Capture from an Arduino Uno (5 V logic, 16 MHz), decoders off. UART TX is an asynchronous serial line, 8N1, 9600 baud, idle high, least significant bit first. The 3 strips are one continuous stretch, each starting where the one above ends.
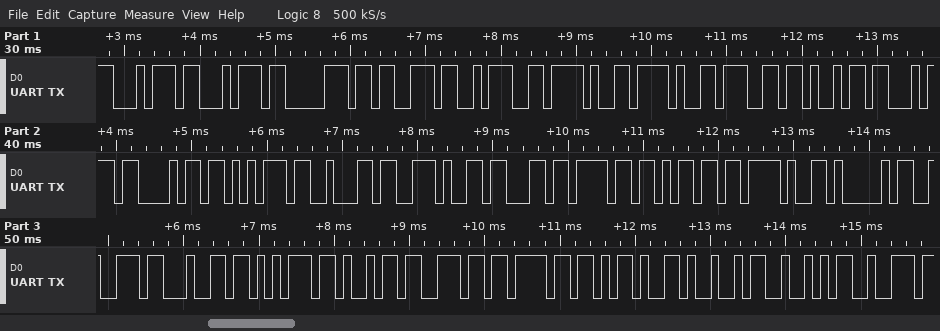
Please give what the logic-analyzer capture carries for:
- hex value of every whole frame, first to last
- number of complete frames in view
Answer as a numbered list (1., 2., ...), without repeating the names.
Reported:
1. 74 74 70 73 3A 2F 2F 67 69 74 68 75 62 2E 63 6F 6D 2F 41 72 64 75 69 6E 6F 2D 49 52 72
2. 29
